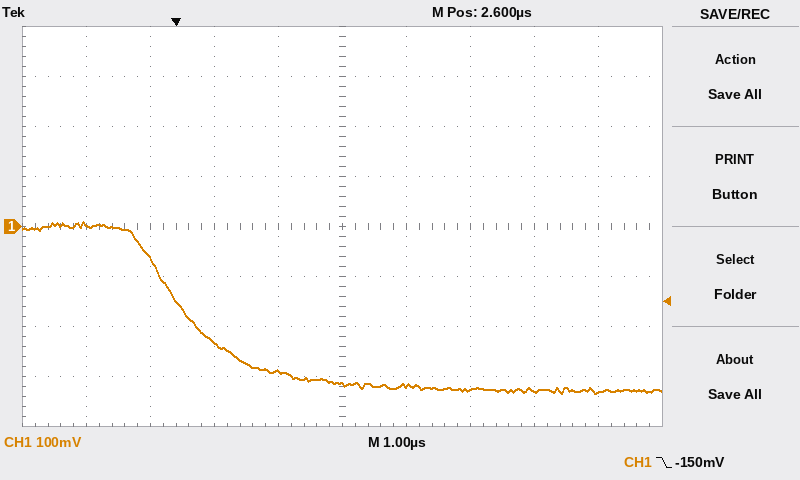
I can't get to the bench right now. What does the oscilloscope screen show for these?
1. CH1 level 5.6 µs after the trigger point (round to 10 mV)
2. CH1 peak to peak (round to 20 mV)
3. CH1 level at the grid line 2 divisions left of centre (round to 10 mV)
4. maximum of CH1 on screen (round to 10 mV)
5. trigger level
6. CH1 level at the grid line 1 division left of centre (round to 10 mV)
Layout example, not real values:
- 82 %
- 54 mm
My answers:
- -330 mV
- 340 mV
- -230 mV
- 10 mV
- -150 mV
- -290 mV
